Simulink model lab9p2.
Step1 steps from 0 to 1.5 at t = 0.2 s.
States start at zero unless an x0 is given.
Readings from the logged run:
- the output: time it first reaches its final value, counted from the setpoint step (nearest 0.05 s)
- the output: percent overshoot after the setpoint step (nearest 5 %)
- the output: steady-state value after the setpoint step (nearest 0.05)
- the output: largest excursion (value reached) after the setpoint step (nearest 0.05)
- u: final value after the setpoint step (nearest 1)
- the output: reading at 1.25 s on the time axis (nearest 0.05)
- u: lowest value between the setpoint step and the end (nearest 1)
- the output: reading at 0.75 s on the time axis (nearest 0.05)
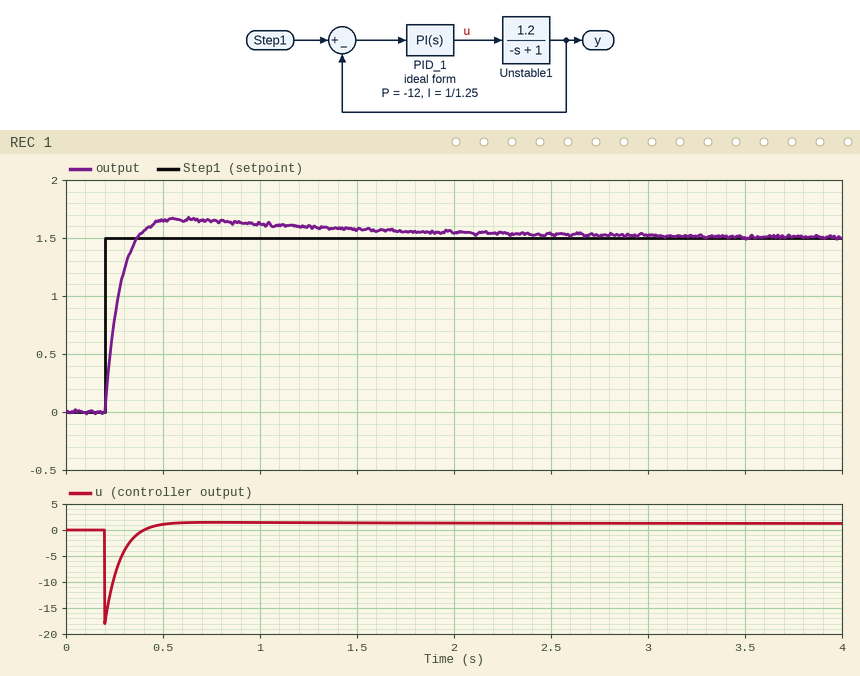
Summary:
0.15 s
10 %
1.50
1.65
1
1.60
-18
1.65
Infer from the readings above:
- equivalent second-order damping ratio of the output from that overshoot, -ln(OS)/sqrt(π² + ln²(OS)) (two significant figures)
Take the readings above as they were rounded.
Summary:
0.59
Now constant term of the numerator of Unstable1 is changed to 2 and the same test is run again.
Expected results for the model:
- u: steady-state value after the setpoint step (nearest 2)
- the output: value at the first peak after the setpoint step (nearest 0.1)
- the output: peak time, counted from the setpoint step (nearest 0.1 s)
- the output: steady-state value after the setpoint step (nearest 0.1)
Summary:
0
1.6
0.3 s
1.5
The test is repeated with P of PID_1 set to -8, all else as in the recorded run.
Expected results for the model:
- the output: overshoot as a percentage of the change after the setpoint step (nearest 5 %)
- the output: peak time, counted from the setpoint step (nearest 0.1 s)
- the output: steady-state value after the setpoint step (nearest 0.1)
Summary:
15 %
0.5 s
1.5
